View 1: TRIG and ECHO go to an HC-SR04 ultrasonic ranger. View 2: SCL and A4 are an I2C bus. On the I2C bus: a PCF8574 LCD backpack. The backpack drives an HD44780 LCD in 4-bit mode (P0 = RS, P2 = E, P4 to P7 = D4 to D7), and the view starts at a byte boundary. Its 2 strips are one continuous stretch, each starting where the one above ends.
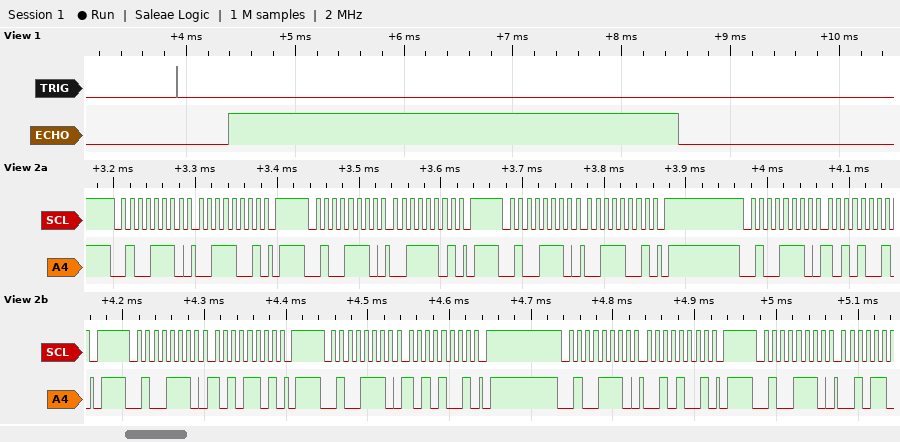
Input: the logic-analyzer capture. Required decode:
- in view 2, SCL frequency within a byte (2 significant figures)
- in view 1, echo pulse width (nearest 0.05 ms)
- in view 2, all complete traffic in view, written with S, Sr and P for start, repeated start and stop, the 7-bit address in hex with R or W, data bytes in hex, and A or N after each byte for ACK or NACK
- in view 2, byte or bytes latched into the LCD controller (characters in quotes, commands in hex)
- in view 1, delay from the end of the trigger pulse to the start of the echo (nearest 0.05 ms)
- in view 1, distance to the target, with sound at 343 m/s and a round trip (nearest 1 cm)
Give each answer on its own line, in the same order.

100 kHz
4.15 ms
S 27W A 39 A P S 27W A 3D A P S 27W A 39 A P S 27W A A9 A P S 27W A AD A P S 27W A A9 A P S 27W A 29 A P S 27W A
':'
0.45 ms
71 cm
